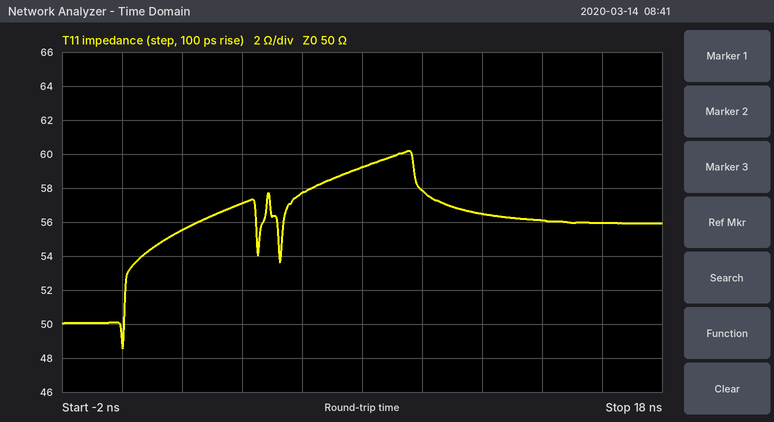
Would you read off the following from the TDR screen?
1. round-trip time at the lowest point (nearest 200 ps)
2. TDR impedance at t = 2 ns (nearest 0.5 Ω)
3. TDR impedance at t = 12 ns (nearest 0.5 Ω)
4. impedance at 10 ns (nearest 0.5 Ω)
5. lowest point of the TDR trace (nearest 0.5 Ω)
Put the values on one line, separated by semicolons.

0.0 ns; 55.5 Ω; 56.5 Ω; 58.0 Ω; 48.5 Ω
